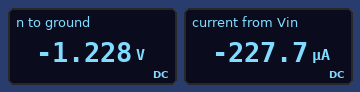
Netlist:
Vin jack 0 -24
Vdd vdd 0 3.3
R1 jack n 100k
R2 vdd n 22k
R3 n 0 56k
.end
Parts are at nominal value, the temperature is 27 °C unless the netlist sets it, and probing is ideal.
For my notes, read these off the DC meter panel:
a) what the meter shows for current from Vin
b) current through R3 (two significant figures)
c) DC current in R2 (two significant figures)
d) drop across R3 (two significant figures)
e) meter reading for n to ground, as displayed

-227.7 µA
22 µA
210 µA
1.2 V
-1.228 V
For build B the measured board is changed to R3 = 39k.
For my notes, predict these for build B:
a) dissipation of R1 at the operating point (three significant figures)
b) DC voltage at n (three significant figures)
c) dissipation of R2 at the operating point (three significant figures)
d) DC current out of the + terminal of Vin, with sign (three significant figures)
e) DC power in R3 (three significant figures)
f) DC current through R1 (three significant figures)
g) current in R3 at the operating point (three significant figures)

5.24 mW
-1.11 V
884 µW
-229 µA
31.6 µW
229 µA
28.5 µA
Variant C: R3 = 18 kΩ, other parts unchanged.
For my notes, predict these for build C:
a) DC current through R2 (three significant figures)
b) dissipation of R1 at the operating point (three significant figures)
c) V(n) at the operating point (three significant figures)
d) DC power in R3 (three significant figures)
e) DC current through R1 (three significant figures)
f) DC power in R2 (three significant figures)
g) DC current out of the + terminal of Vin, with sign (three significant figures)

187 µA
5.38 mW
-811 mV
36.5 µW
232 µA
768 µW
-232 µA
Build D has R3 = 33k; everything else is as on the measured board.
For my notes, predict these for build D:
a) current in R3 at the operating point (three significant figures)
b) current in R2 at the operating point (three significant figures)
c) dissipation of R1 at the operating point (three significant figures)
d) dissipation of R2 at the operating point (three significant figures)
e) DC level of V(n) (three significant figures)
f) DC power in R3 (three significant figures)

31.8 µA
198 µA
5.27 mW
860 µW
-1.05 V
33.4 µW
